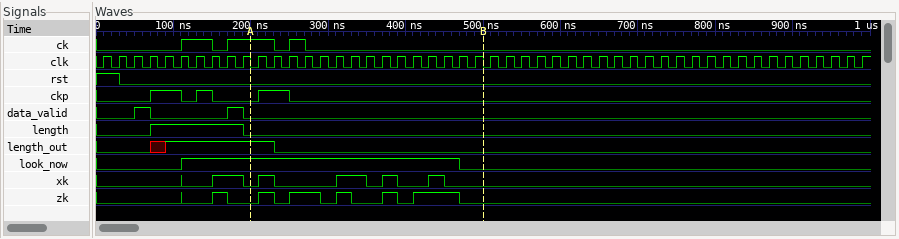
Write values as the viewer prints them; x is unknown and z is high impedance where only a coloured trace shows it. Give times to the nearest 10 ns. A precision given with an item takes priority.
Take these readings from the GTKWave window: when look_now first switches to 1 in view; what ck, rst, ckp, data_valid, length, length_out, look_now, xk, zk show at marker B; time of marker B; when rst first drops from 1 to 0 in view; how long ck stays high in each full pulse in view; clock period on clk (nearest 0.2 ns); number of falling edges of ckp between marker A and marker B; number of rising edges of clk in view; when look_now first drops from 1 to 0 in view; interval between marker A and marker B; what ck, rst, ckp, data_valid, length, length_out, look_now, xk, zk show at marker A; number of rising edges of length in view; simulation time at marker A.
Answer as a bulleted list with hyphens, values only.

- 110 ns
- ck=0, rst=0, ckp=0, data_valid=0, length=0, length_out=0, look_now=0, xk=0, zk=0
- 500 ns
- 30 ns
- 40 ns, 60 ns, 20 ns
- 20 ns
- 1
- 50
- 470 ns
- 300 ns
- ck=1, rst=0, ckp=0, data_valid=0, length=0, length_out=1, look_now=1, xk=0, zk=0
- 1
- 200 ns
